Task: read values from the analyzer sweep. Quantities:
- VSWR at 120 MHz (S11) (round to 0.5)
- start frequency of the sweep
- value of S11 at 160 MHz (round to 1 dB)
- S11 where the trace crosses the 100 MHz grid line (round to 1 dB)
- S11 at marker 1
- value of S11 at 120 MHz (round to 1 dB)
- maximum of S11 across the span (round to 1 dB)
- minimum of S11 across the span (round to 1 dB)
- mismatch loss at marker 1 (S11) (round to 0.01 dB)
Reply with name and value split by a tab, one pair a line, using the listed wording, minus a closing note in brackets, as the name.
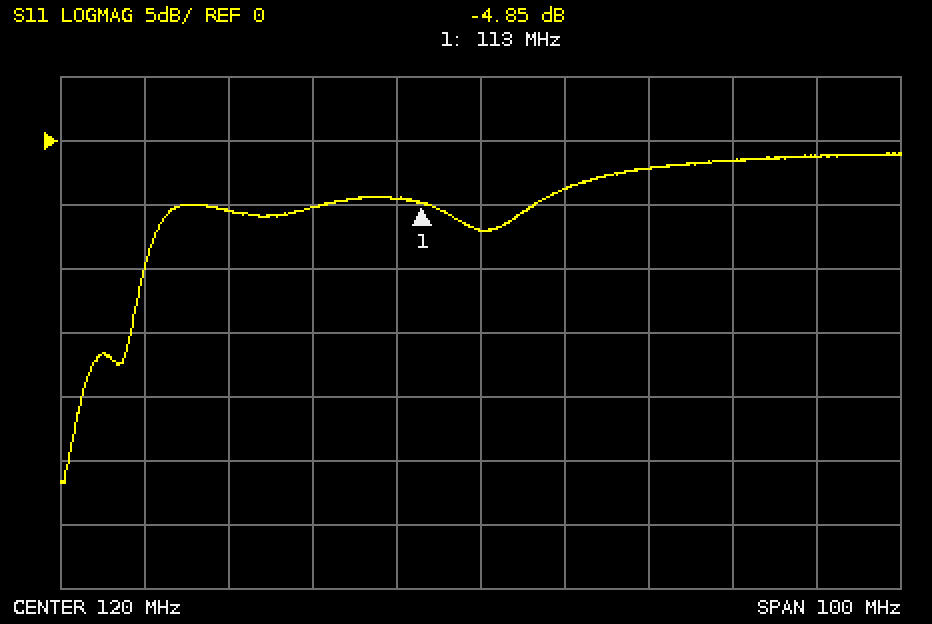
VSWR at 120 MHz (S11)	2.5
start frequency of the sweep	70 MHz
value of S11 at 160 MHz	-1 dB
S11 where the trace crosses the 100 MHz grid line	-5 dB
S11 at marker 1	-4.85 dB
value of S11 at 120 MHz	-7 dB
maximum of S11 across the span	-1 dB
minimum of S11 across the span	-27 dB
mismatch loss at marker 1 (S11)	1.72 dB
